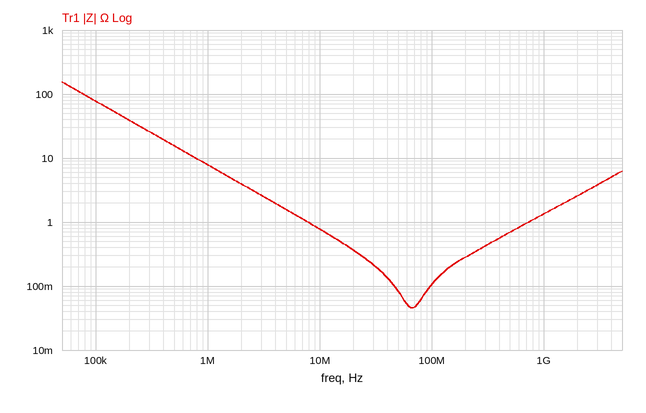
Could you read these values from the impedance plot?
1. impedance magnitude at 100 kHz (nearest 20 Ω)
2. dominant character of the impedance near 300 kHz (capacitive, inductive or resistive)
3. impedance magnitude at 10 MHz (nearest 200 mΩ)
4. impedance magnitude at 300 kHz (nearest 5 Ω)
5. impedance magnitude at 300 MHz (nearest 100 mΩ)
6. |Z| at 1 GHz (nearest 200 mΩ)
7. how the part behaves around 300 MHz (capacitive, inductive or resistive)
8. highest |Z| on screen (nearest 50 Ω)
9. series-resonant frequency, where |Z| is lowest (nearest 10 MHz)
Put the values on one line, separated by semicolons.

80 Ω; capacitive; 800 mΩ; 25 Ω; 400 mΩ; 1.4 Ω; inductive; 150 Ω; 70 MHz
